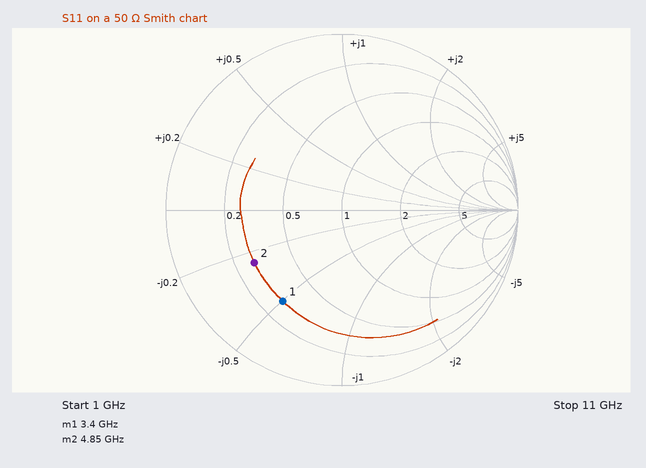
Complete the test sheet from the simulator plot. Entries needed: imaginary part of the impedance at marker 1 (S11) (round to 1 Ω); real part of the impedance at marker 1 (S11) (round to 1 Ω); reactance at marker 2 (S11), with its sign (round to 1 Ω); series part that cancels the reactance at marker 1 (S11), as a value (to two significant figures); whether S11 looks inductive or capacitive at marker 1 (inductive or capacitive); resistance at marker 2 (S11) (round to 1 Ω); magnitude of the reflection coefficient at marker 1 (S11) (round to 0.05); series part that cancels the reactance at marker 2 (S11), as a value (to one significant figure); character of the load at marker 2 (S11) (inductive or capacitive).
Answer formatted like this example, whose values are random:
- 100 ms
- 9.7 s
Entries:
- -25 Ω
- 15 Ω
- -13 Ω
- 1.2 nH
- capacitive
- 14 Ω
- 0.60
- 400 pH
- capacitive
